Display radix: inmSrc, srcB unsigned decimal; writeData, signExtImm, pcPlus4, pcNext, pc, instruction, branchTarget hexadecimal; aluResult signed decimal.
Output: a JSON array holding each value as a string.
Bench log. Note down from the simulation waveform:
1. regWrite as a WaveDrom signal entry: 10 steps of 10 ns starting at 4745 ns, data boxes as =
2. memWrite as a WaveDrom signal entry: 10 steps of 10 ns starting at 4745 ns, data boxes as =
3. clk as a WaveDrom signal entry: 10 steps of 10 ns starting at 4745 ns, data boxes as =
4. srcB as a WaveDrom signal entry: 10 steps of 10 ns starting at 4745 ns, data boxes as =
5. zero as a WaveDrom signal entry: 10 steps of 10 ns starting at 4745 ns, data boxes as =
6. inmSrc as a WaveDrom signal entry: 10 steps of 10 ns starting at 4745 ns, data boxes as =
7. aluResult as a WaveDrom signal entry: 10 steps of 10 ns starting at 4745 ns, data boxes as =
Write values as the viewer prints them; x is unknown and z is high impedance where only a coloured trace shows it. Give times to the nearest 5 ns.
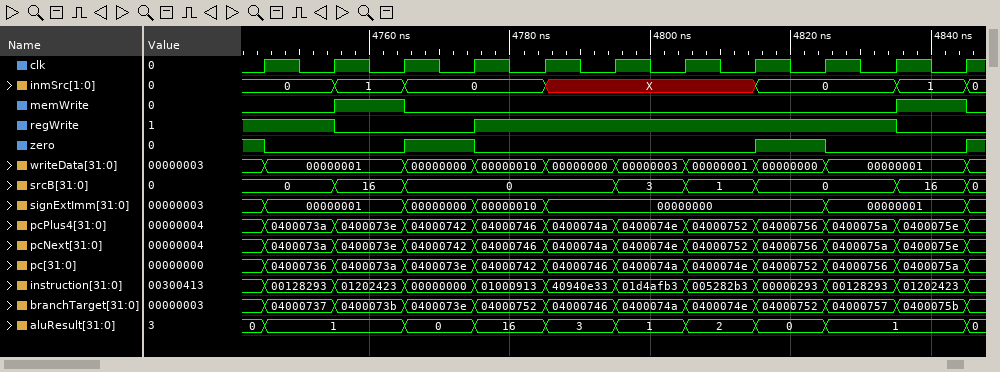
["{name: 'regWrite', wave: '10.1.....0'}", "{name: 'memWrite', wave: '010......1'}", "{name: 'clk', wave: 'p.........'}", "{name: 'srcB', wave: '===..===.=', data: '0 16 0 3 1 0 16'}", "{name: 'zero', wave: '0.10...10.'}", "{name: 'inmSrc', wave: '===.x..=.=', data: '0 1 0 0 1'}", "{name: 'aluResult', wave: '=.=======.', data: '1 0 16 3 1 2 0 1'}"]
